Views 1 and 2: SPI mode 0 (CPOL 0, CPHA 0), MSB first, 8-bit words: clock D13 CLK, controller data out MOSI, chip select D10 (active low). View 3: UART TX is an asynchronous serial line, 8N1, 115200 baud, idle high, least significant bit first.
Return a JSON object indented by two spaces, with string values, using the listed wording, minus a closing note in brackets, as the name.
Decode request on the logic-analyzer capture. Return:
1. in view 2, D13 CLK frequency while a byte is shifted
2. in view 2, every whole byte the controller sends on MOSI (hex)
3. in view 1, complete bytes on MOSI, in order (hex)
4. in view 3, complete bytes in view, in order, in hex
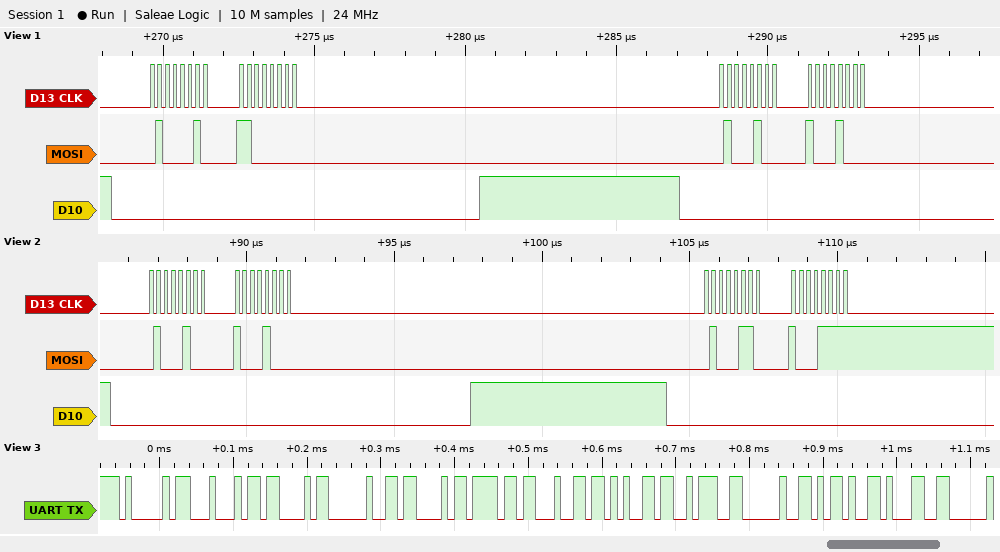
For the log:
{
  "in view 2, D13 CLK frequency while a byte is shifted": "4 MHz",
  "in view 2, every whole byte the controller sends on MOSI": "44 88 46 8F",
  "in view 1, complete bytes on MOSI, in order": "42 C0 44 88",
  "in view 3, complete bytes in view, in order, in hex": "41 44 43 20 43 6F 64 65 3A 20 2D 31"
}
